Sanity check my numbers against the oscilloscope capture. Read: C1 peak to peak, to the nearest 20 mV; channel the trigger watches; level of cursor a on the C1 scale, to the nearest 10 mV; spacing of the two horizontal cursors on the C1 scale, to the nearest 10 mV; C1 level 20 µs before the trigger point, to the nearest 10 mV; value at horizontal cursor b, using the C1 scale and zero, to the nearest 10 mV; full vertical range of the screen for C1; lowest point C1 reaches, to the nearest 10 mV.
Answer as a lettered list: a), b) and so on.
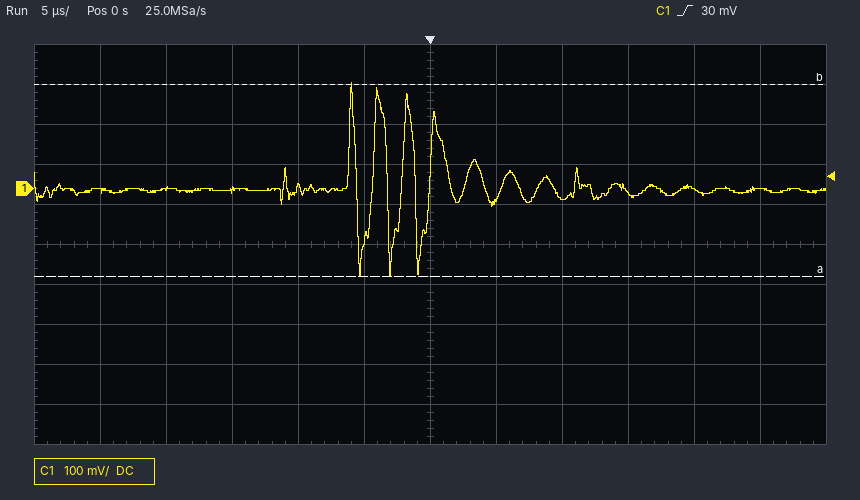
a) 480 mV
b) C1
c) -220 mV
d) 480 mV
e) 0 mV
f) 260 mV
g) 1 V
h) -220 mV
